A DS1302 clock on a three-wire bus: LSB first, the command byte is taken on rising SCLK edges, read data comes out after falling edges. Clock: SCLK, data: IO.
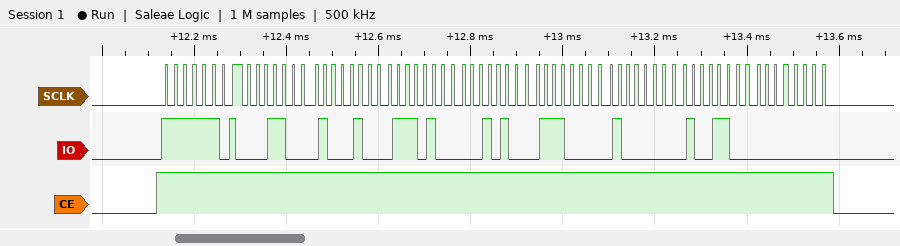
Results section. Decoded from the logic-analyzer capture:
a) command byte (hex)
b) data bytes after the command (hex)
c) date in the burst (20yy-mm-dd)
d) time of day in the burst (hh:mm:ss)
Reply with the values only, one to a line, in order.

0xBF
18 11 17 14 07 01 19 00
2019-07-14
17:11:18
